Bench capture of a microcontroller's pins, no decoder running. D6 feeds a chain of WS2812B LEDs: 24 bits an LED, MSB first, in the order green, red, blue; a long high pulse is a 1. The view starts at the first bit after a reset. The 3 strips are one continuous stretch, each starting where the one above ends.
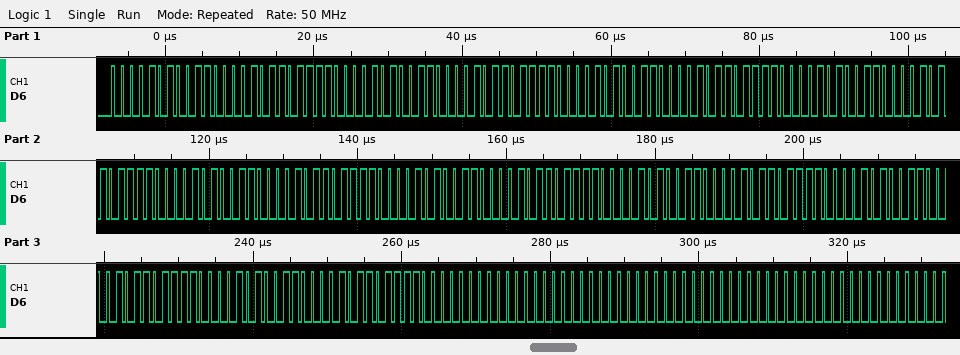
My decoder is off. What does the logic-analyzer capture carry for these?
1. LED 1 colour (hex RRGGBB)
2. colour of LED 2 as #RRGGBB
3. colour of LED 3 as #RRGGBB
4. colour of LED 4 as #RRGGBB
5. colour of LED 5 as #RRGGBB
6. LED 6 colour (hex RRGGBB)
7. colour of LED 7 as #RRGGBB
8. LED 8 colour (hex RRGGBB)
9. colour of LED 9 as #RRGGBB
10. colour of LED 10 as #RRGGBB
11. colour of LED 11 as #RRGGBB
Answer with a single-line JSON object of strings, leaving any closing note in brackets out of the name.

{"LED 1 colour": "#610A6F", "colour of LED 2 as #RRGGBB": "#610A6F", "colour of LED 3 as #RRGGBB": "#610A6F", "colour of LED 4 as #RRGGBB": "#610A6F", "colour of LED 5 as #RRGGBB": "#610A6F", "LED 6 colour": "#610A6F", "colour of LED 7 as #RRGGBB": "#610A6F", "LED 8 colour": "#610A6F", "colour of LED 9 as #RRGGBB": "#610A6F", "colour of LED 10 as #RRGGBB": "#000000", "colour of LED 11 as #RRGGBB": "#000000"}
